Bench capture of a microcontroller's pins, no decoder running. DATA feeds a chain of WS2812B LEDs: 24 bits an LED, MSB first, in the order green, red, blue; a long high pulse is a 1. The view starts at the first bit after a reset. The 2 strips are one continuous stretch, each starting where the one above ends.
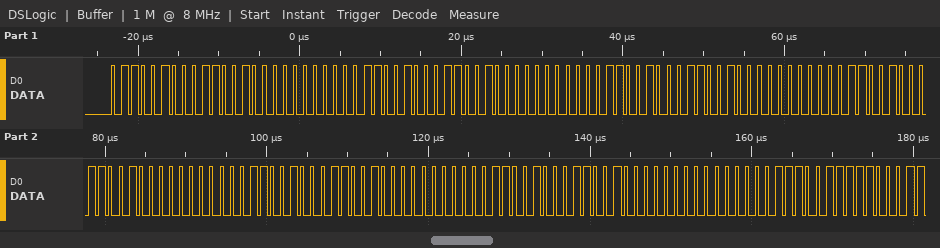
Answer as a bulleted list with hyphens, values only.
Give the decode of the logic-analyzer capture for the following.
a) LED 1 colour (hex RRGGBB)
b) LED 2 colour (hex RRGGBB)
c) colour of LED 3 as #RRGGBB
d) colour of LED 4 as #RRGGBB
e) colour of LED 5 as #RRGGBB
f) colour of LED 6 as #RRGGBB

- #646400
- #646400
- #646400
- #646400
- #646400
- #646400
